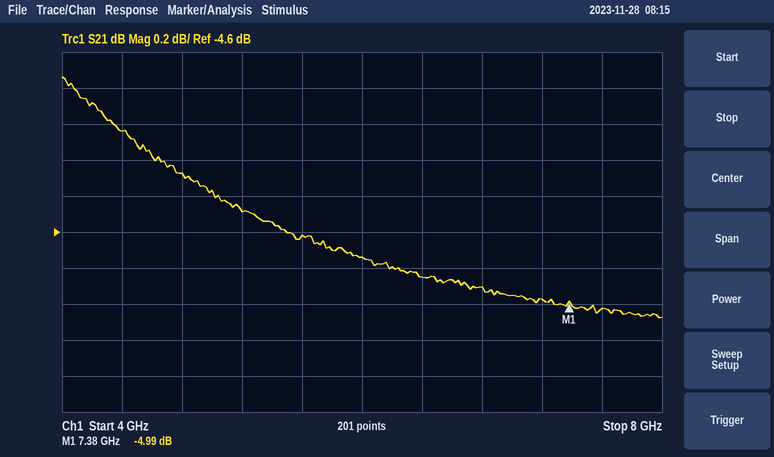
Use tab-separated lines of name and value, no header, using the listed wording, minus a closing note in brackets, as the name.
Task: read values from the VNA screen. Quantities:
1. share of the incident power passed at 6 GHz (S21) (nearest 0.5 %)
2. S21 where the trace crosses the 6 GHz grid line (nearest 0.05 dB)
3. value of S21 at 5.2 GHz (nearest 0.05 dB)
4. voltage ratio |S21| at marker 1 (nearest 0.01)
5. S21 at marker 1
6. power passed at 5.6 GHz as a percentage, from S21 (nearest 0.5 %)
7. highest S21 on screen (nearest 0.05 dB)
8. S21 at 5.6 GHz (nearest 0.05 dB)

share of the incident power passed at 6 GHz (S21)	33.5 %
S21 where the trace crosses the 6 GHz grid line	-4.75 dB
value of S21 at 5.2 GHz	-4.50 dB
voltage ratio |S21| at marker 1	0.56
S21 at marker 1	-4.99 dB
power passed at 5.6 GHz as a percentage, from S21	34.5 %
highest S21 on screen	-3.75 dB
S21 at 5.6 GHz	-4.60 dB
